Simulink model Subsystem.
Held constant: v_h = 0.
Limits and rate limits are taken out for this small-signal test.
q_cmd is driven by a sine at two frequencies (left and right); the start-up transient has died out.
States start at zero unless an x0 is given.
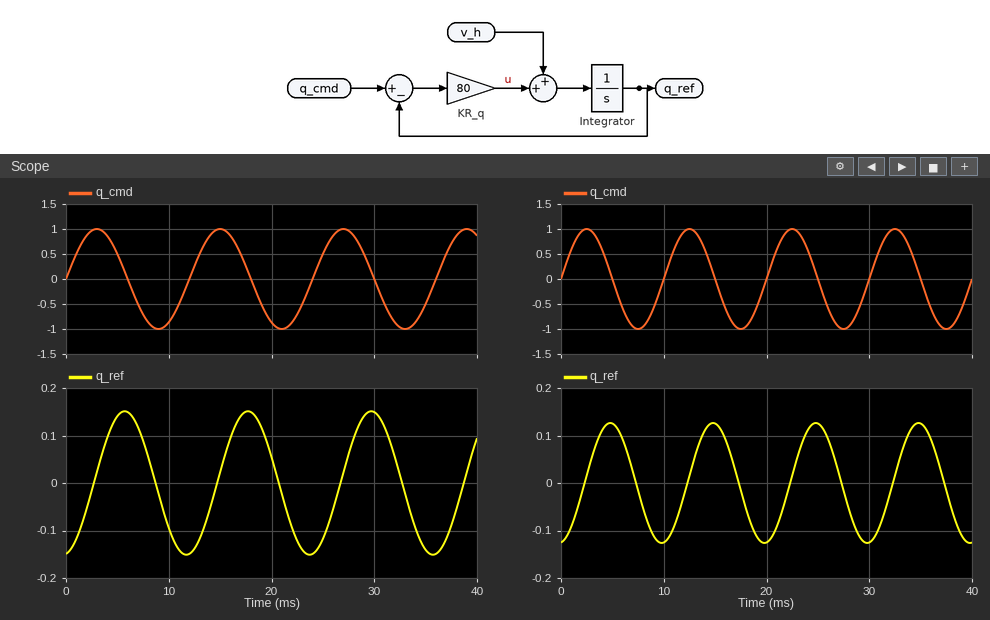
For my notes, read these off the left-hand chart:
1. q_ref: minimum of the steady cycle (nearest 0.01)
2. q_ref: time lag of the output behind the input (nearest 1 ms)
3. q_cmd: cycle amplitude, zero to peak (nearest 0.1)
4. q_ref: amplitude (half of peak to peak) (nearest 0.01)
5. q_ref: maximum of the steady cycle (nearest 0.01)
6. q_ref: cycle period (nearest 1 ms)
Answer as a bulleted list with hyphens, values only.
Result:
- -0.15
- 3 ms
- 1.0
- 0.15
- 0.15
- 12 ms
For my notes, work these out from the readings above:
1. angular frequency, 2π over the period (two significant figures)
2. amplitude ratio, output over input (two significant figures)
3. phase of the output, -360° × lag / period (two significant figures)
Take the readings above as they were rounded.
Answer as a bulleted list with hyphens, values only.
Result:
- 0.52 rad/ms
- 0.15
- -90°
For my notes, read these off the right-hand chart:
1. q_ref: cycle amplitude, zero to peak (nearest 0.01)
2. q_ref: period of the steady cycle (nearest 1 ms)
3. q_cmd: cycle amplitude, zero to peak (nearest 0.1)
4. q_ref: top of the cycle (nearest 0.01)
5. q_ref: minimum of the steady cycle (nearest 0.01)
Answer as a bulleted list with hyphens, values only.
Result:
- 0.13
- 10 ms
- 1.0
- 0.13
- -0.13
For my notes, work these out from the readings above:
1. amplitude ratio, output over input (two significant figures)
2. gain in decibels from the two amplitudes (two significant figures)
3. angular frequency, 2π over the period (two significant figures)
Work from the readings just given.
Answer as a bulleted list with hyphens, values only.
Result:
- 0.13
- -18 dB
- 0.63 rad/ms
